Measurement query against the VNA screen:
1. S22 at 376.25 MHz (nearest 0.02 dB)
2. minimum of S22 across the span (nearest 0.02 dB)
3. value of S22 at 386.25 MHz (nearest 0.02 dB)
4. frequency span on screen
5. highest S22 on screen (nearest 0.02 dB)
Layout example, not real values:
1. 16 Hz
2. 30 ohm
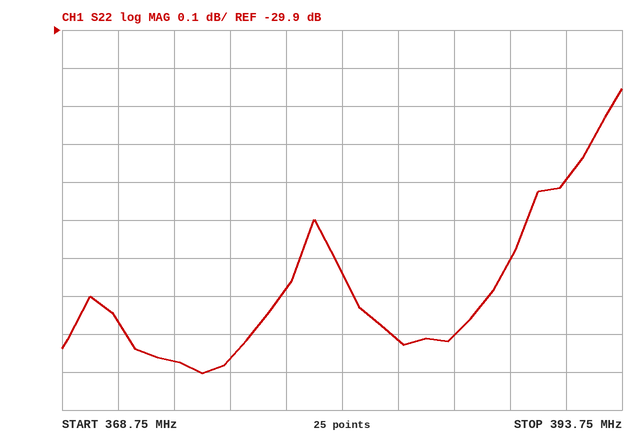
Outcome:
1. -30.76 dB
2. -30.80 dB
3. -30.70 dB
4. 25 MHz
5. -30.06 dB
